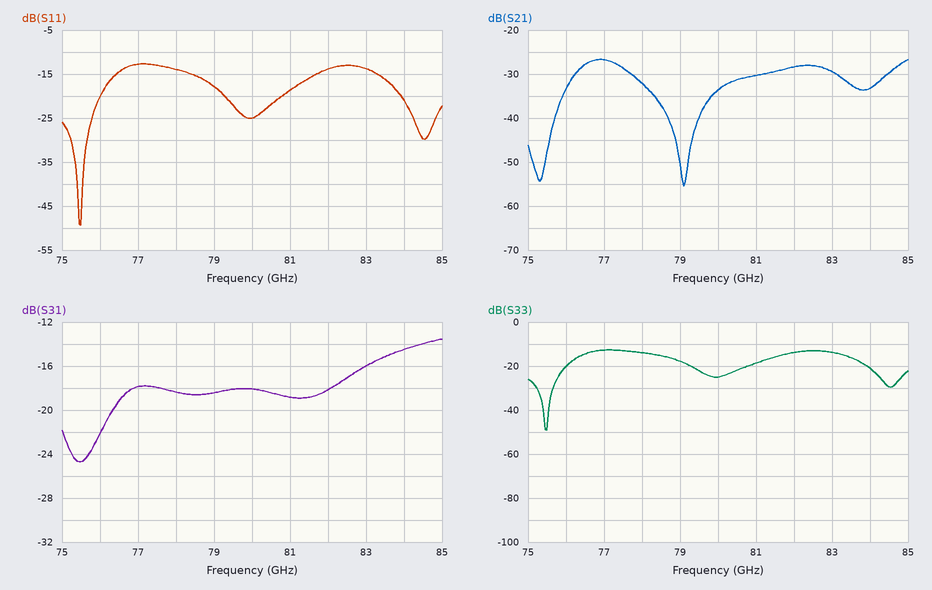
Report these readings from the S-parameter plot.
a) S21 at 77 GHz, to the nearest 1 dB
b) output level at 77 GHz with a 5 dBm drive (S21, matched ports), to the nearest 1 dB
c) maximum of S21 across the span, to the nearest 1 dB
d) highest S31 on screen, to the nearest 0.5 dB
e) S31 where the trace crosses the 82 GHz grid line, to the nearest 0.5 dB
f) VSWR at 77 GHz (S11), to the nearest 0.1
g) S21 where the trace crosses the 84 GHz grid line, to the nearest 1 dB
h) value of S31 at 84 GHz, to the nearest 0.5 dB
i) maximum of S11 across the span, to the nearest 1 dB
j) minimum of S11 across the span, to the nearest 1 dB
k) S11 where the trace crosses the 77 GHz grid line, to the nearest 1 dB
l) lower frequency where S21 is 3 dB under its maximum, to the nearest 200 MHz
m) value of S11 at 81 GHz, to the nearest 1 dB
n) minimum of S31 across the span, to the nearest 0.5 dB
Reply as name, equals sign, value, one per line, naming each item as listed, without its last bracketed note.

S21 at 77 GHz, to the nearest 1 dB = -27 dB
output level at 77 GHz with a 5 dBm drive (S21, matched ports), to the nearest 1 dB = -22 dBm
maximum of S21 across the span, to the nearest 1 dB = -27 dB
highest S31 on screen, to the nearest 0.5 dB = -13.5 dB
S31 where the trace crosses the 82 GHz grid line, to the nearest 0.5 dB = -18.0 dB
VSWR at 77 GHz (S11), to the nearest 0.1 = 1.6
S21 where the trace crosses the 84 GHz grid line, to the nearest 1 dB = -33 dB
value of S31 at 84 GHz, to the nearest 0.5 dB = -14.5 dB
maximum of S11 across the span, to the nearest 1 dB = -13 dB
minimum of S11 across the span, to the nearest 1 dB = -49 dB
S11 where the trace crosses the 77 GHz grid line, to the nearest 1 dB = -13 dB
lower frequency where S21 is 3 dB under its maximum, to the nearest 200 MHz = 76.2 GHz
value of S11 at 81 GHz, to the nearest 1 dB = -19 dB
minimum of S31 across the span, to the nearest 0.5 dB = -24.5 dB
